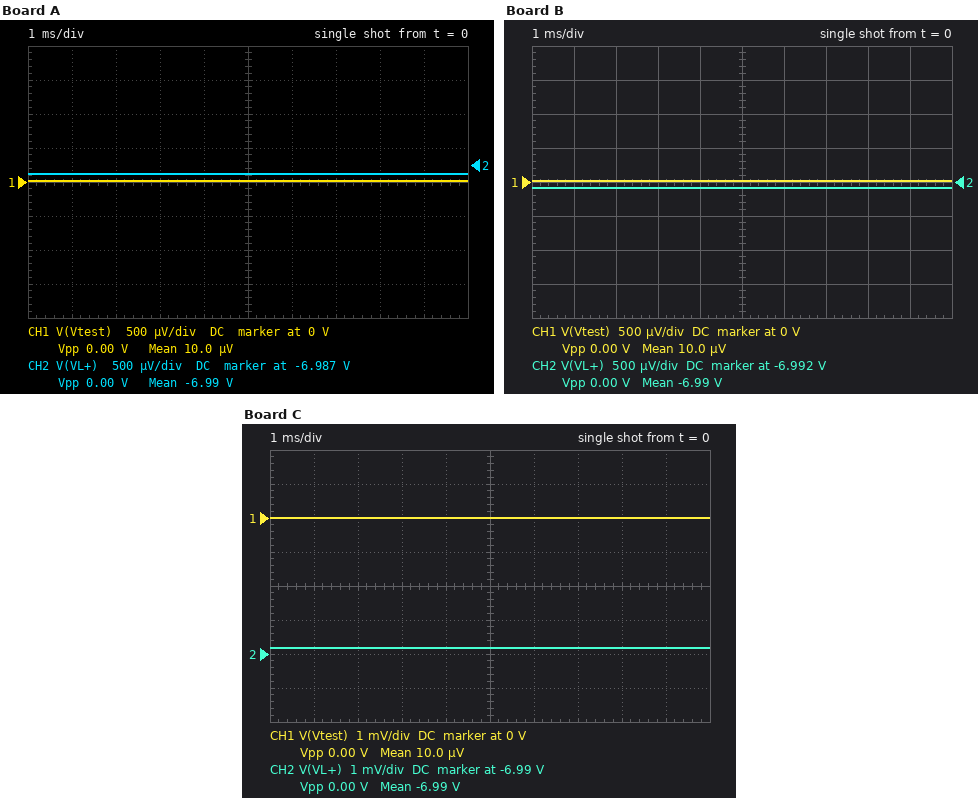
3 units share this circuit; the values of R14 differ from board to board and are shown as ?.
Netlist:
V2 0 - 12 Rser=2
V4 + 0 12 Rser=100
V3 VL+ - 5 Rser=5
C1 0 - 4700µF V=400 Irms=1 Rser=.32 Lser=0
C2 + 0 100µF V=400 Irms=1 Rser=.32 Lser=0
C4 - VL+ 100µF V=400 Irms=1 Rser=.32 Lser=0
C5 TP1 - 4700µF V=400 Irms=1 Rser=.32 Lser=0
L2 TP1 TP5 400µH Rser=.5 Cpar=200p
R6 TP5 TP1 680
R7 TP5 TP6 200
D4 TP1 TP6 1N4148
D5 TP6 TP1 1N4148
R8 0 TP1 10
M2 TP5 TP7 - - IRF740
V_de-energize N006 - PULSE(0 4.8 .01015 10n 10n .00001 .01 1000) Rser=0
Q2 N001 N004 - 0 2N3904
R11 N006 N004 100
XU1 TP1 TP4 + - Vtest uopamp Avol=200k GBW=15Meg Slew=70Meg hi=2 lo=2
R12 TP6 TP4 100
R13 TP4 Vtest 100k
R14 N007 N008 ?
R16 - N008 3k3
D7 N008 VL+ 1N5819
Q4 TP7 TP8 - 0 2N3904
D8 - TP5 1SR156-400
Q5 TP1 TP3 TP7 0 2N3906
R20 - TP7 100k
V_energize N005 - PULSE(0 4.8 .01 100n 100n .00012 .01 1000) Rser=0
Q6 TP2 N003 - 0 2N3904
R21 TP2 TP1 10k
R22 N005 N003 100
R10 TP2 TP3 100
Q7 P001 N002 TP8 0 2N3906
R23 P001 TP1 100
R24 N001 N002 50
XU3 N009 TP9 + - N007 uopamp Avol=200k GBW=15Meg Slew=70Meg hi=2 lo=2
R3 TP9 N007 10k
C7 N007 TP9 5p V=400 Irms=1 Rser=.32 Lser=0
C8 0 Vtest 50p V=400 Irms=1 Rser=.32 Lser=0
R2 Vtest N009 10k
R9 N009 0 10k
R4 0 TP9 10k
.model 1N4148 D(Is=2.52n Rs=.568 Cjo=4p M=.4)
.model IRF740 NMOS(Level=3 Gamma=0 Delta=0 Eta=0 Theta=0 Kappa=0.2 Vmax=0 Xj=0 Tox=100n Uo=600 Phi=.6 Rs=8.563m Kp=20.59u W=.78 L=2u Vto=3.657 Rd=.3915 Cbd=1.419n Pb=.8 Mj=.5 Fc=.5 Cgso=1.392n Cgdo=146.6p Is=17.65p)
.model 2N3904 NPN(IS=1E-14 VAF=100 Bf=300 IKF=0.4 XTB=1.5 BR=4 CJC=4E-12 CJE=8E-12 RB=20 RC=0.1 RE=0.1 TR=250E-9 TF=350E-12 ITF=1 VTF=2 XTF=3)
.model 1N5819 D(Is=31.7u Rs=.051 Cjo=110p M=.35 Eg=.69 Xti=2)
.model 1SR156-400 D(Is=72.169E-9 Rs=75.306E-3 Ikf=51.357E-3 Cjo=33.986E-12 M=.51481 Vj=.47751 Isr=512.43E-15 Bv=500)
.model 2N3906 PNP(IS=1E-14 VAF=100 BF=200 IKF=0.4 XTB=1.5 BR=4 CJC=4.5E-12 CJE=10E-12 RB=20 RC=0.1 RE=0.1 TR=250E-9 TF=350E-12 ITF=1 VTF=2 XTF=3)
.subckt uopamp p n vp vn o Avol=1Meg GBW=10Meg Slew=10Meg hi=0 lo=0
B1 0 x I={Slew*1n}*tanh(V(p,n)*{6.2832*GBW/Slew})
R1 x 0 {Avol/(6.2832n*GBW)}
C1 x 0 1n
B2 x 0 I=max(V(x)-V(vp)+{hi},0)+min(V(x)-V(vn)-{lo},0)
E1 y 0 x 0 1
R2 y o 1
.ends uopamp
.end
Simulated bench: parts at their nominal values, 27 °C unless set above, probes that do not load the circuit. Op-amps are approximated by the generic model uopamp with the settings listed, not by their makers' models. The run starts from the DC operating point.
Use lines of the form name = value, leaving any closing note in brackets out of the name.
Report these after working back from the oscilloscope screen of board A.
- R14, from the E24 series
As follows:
R14, from the E24 series = 2.4 kΩ
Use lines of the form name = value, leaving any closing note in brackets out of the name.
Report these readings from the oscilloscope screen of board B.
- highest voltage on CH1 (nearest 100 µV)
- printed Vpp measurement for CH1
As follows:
highest voltage on CH1 = 0 V
printed Vpp measurement for CH1 = 0.00 V
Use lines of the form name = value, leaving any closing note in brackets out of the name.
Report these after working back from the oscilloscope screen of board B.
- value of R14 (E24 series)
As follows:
value of R14 = 3 kΩ
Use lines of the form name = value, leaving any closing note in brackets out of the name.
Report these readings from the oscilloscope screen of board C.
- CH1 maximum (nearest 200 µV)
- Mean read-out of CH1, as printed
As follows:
CH1 maximum = 0 V
Mean read-out of CH1, as printed = 10.0 µV
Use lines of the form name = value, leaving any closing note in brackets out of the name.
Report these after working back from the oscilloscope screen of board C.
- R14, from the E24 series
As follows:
R14, from the E24 series = 2.7 kΩ
